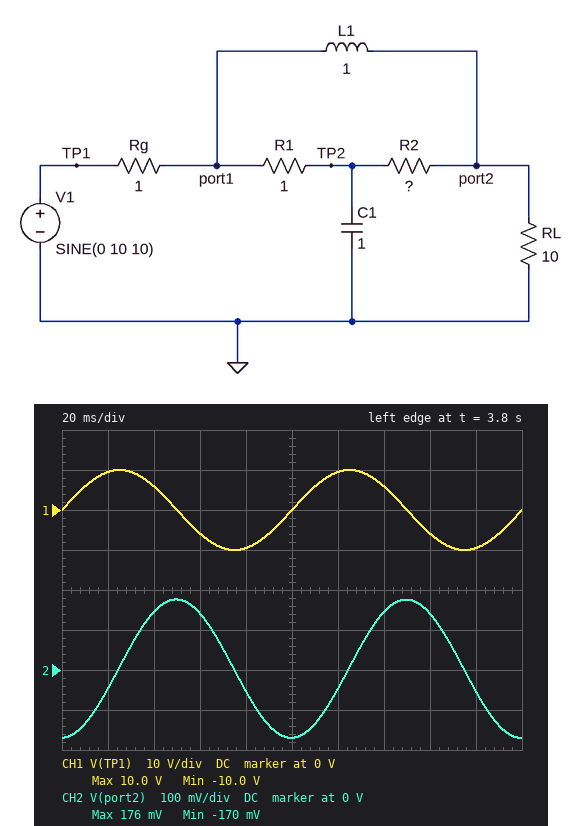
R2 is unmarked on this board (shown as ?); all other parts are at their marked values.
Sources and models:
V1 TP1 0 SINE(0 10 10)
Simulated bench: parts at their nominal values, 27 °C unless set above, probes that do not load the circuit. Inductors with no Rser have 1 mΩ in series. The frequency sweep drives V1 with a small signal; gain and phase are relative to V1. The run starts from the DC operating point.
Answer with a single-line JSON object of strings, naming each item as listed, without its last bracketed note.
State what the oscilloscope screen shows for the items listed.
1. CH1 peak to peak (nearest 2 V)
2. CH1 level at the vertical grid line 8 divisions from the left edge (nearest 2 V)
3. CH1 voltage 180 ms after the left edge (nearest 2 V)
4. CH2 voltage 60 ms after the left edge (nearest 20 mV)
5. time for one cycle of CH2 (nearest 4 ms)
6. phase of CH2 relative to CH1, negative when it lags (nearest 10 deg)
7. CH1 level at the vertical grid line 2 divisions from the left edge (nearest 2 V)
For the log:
{"CH1 peak to peak": "20 V", "CH1 level at the vertical grid line 8 divisions from the left edge": "-6 V", "CH1 voltage 180 ms after the left edge": "-10 V", "CH2 voltage 60 ms after the left edge": "140 mV", "time for one cycle of CH2": "100 ms", "phase of CH2 relative to CH1, negative when it lags": "-90 deg", "CH1 level at the vertical grid line 2 divisions from the left edge": "6 V"}
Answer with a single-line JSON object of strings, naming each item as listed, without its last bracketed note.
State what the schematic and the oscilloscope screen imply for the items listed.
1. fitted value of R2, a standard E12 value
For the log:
{"fitted value of R2, a standard E12 value": "1.5 Ω"}
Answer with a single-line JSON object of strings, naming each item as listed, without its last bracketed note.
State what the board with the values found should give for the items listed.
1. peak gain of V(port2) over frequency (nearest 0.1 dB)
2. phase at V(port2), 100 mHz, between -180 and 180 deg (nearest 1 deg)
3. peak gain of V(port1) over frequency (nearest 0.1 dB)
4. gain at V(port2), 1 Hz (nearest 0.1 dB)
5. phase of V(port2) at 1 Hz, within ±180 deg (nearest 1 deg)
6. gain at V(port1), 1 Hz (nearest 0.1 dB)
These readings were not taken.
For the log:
{"peak gain of V(port2) over frequency": "-0.8 dB", "phase at V(port2), 100 mHz, between -180 and 180 deg": "-30 deg", "peak gain of V(port1) over frequency": "-0.8 dB", "gain at V(port2), 1 Hz": "-15.5 dB", "phase of V(port2) at 1 Hz, within ±180 deg": "-78 deg", "gain at V(port1), 1 Hz": "-6.2 dB"}
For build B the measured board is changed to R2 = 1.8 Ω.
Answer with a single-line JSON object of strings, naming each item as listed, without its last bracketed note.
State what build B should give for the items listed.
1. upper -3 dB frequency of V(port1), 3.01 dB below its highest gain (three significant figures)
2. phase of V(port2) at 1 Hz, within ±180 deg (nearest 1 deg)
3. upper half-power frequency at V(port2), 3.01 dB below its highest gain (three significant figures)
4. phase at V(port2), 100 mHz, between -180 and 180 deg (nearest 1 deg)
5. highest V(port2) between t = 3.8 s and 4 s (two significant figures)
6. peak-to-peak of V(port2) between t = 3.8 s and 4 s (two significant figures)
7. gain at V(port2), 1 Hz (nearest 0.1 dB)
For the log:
{"upper -3 dB frequency of V(port1), 3.01 dB below its highest gain": "117 mHz", "phase of V(port2) at 1 Hz, within ±180 deg": "-76 deg", "upper half-power frequency at V(port2), 3.01 dB below its highest gain": "156 mHz", "phase at V(port2), 100 mHz, between -180 and 180 deg": "-29 deg", "highest V(port2) between t = 3.8 s and 4 s": "190 mV", "peak-to-peak of V(port2) between t = 3.8 s and 4 s": "380 mV", "gain at V(port2), 1 Hz": "-14.8 dB"}
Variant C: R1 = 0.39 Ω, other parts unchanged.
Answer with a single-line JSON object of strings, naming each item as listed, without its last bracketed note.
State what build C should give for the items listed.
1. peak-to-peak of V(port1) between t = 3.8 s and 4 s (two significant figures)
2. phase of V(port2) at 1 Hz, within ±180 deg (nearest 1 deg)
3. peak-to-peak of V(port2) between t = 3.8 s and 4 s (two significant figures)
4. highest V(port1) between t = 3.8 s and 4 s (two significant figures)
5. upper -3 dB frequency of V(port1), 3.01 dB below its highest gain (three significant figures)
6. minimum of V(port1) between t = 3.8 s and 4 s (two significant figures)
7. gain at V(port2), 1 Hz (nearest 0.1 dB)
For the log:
{"peak-to-peak of V(port1) between t = 3.8 s and 4 s": "5.6 V", "phase of V(port2) at 1 Hz, within ±180 deg": "-79 deg", "peak-to-peak of V(port2) between t = 3.8 s and 4 s": "320 mV", "highest V(port1) between t = 3.8 s and 4 s": "2.8 V", "upper -3 dB frequency of V(port1), 3.01 dB below its highest gain": "136 mHz", "minimum of V(port1) between t = 3.8 s and 4 s": "-2.8 V", "gain at V(port2), 1 Hz": "-16.2 dB"}
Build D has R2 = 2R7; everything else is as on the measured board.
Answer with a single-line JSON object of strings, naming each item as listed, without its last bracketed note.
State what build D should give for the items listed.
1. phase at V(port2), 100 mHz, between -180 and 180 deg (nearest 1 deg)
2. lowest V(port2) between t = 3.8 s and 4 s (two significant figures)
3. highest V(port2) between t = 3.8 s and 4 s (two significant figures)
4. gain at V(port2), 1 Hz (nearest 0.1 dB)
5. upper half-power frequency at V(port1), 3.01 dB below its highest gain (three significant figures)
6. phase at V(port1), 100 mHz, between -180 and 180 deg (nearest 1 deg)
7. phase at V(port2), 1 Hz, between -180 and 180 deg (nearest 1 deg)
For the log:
{"phase at V(port2), 100 mHz, between -180 and 180 deg": "-27 deg", "lowest V(port2) between t = 3.8 s and 4 s": "-230 mV", "highest V(port2) between t = 3.8 s and 4 s": "240 mV", "gain at V(port2), 1 Hz": "-13.3 dB", "upper half-power frequency at V(port1), 3.01 dB below its highest gain": "119 mHz", "phase at V(port1), 100 mHz, between -180 and 180 deg": "-20 deg", "phase at V(port2), 1 Hz, between -180 and 180 deg": "-71 deg"}
